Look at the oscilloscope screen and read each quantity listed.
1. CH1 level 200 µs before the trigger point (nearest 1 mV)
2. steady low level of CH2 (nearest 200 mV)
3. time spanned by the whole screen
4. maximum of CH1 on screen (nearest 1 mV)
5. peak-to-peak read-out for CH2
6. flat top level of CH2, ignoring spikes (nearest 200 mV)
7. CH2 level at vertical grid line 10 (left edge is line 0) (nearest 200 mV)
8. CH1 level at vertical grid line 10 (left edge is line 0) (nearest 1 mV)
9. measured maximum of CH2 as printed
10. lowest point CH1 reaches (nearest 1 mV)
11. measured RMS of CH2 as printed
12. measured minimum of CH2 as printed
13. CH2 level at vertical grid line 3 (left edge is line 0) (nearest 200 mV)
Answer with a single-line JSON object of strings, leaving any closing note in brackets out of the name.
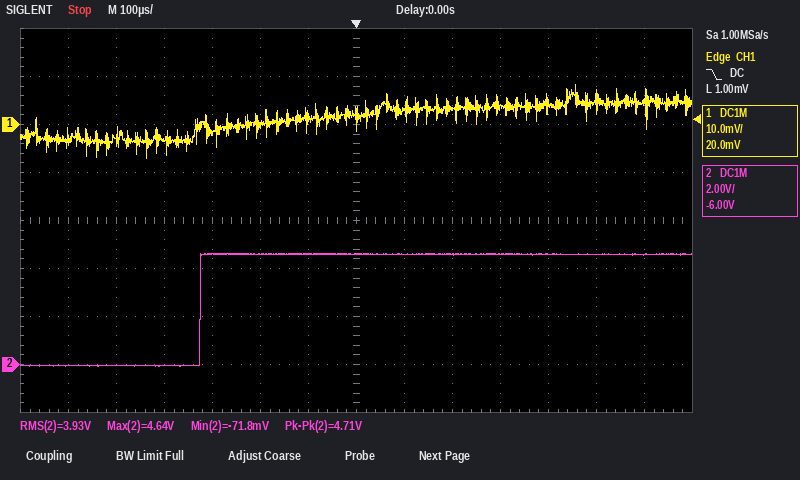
{"CH1 level 200 µs before the trigger point": "0 mV", "steady low level of CH2": "0.0 V", "time spanned by the whole screen": "1.4 ms", "maximum of CH1 on screen": "8 mV", "peak-to-peak read-out for CH2": "4.71 V", "flat top level of CH2, ignoring spikes": "4.6 V", "CH2 level at vertical grid line 10 (left edge is line 0)": "4.6 V", "CH1 level at vertical grid line 10 (left edge is line 0)": "4 mV", "measured maximum of CH2 as printed": "4.64 V", "lowest point CH1 reaches": "-7 mV", "measured RMS of CH2 as printed": "3.93 V", "measured minimum of CH2 as printed": "-71.8 mV", "CH2 level at vertical grid line 3 (left edge is line 0)": "0.0 V"}
